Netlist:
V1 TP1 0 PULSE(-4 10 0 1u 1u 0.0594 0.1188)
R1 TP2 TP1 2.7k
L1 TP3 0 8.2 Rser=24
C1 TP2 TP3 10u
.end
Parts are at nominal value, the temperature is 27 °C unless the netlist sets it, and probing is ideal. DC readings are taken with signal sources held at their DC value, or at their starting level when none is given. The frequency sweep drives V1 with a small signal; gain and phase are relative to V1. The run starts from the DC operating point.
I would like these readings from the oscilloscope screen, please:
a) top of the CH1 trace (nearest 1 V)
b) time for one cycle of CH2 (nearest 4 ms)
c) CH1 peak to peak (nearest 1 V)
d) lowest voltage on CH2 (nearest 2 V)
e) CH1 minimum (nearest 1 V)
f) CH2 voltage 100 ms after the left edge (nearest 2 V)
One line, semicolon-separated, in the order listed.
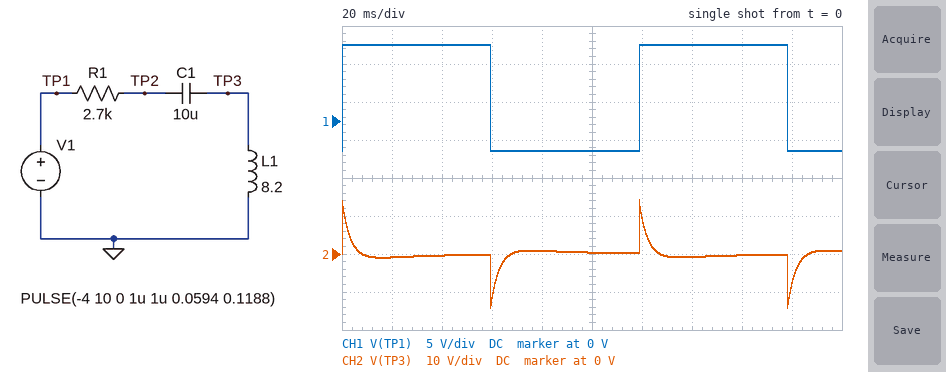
10 V; 120 ms; 14 V; -14 V; -4 V; 0 V
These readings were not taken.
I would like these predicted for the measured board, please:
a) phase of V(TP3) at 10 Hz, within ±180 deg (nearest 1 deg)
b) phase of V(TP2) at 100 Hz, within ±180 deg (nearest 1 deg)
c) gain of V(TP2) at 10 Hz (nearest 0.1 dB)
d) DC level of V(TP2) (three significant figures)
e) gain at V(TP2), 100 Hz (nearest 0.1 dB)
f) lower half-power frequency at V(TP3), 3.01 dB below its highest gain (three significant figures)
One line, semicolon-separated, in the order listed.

109 deg; 28 deg; -8.7 dB; -4.00 V; -1.1 dB; 47.1 Hz
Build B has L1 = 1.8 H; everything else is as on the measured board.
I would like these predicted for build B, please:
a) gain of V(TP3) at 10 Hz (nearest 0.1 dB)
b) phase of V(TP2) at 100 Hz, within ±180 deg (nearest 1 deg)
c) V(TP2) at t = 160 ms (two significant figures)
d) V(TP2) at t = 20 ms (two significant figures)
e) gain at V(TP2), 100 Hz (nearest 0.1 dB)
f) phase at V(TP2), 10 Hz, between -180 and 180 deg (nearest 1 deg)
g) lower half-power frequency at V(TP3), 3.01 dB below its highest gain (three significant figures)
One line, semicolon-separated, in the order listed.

-28.6 dB; 69 deg; 7.2 V; 3.1 V; -9.5 dB; -61 deg; 235 Hz
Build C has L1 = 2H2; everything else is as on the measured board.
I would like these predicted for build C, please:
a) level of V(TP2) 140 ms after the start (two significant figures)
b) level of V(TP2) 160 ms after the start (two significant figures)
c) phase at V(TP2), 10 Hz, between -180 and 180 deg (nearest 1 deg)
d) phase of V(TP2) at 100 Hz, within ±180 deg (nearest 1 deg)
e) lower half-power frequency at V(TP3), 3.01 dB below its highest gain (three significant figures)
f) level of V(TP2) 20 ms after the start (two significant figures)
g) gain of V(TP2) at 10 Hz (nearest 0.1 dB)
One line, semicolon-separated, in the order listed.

4.0 V; 7.2 V; -61 deg; 65 deg; 191 Hz; 3.1 V; -6.5 dB
